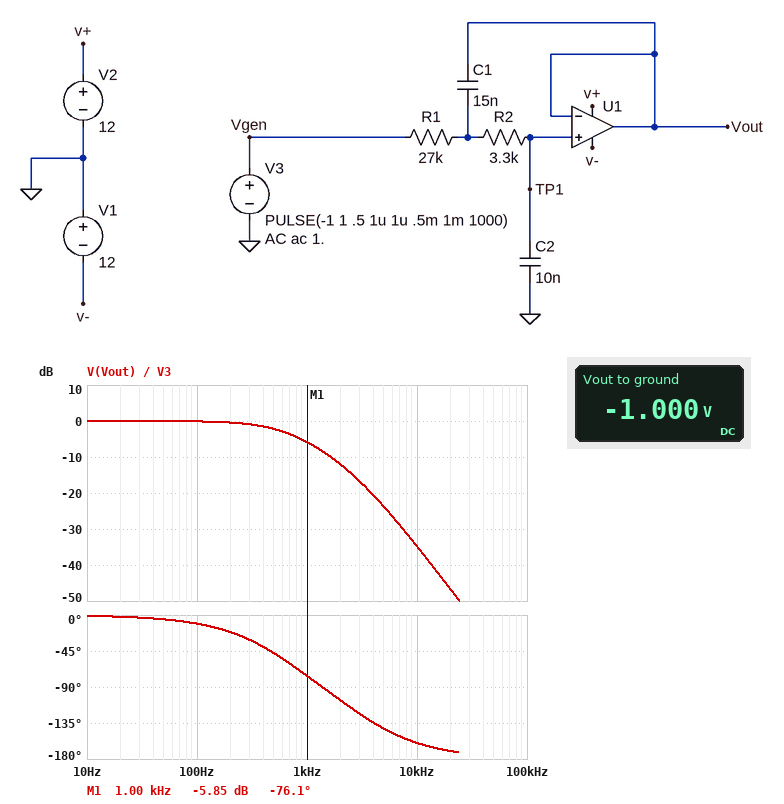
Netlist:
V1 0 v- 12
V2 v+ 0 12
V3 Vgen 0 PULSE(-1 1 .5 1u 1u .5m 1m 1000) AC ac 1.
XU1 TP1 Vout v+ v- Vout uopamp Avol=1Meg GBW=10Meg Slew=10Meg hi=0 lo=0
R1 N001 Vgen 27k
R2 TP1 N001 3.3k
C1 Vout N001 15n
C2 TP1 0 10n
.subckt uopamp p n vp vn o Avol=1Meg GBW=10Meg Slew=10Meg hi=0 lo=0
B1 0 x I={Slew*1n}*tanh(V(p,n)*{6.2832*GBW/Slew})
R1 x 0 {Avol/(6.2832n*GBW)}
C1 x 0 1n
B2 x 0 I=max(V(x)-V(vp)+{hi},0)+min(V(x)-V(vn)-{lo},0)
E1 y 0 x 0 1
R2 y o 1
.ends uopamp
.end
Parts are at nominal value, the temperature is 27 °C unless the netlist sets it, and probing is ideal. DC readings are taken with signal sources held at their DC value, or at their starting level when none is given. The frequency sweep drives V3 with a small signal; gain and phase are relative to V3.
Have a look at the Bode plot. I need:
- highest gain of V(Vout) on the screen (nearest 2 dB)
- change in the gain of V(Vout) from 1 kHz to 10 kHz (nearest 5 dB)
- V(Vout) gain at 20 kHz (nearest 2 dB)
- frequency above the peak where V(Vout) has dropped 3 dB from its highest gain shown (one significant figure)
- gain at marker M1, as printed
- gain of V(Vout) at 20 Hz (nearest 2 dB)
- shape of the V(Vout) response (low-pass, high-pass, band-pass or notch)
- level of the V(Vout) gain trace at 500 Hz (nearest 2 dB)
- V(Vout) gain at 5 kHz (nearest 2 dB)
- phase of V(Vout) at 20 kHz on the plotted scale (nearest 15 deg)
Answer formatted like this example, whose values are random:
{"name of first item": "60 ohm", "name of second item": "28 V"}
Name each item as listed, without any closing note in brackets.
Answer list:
{"highest gain of V(Vout) on the screen": "0 dB", "change in the gain of V(Vout) from 1 kHz to 10 kHz": "-30 dB", "V(Vout) gain at 20 kHz": "-46 dB", "frequency above the peak where V(Vout) has dropped 3 dB from its highest gain shown": "600 Hz", "gain at marker M1, as printed": "-5.85 dB", "gain of V(Vout) at 20 Hz": "0 dB", "shape of the V(Vout) response": "low-pass", "level of the V(Vout) gain trace at 500 Hz": "-2 dB", "V(Vout) gain at 5 kHz": "-24 dB", "phase of V(Vout) at 20 kHz on the plotted scale": "-165 deg"}
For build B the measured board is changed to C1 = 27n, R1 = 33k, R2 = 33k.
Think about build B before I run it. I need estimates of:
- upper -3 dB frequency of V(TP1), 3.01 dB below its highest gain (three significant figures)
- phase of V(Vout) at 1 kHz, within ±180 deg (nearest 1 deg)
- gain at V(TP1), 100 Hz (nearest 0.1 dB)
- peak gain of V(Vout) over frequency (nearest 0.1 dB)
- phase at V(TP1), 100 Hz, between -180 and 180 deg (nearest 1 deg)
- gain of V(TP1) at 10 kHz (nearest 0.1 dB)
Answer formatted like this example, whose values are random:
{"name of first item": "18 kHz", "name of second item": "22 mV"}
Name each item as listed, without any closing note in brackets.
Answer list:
{"upper -3 dB frequency of V(TP1), 3.01 dB below its highest gain": "325 Hz", "phase of V(Vout) at 1 kHz, within ±180 deg": "-159 deg", "gain at V(TP1), 100 Hz": "0.2 dB", "peak gain of V(Vout) over frequency": "0.3 dB", "phase at V(TP1), 100 Hz, between -180 and 180 deg": "-25 deg", "gain of V(TP1) at 10 kHz": "-61.3 dB"}
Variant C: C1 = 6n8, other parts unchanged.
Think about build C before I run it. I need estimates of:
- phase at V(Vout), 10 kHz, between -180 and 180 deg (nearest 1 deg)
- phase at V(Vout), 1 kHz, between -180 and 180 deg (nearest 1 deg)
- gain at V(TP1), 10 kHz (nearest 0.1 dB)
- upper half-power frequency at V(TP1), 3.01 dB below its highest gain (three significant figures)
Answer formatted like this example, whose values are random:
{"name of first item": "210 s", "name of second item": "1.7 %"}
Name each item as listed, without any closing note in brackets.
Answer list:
{"phase at V(Vout), 10 kHz, between -180 and 180 deg": "-140 deg", "phase at V(Vout), 1 kHz, between -180 and 180 deg": "-68 deg", "gain at V(TP1), 10 kHz": "-29.5 dB", "upper half-power frequency at V(TP1), 3.01 dB below its highest gain": "562 Hz"}
